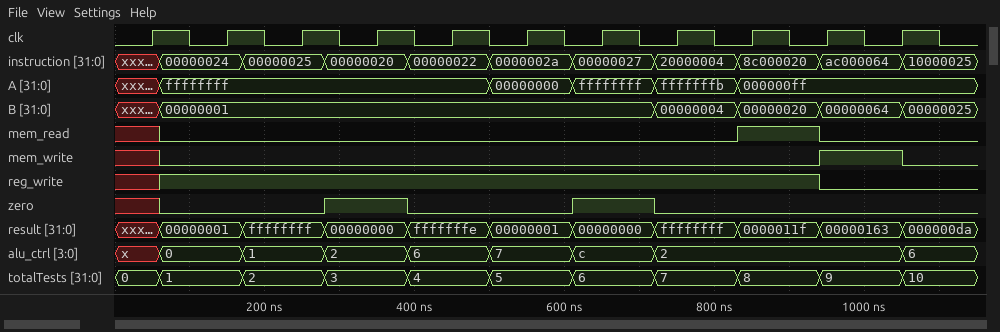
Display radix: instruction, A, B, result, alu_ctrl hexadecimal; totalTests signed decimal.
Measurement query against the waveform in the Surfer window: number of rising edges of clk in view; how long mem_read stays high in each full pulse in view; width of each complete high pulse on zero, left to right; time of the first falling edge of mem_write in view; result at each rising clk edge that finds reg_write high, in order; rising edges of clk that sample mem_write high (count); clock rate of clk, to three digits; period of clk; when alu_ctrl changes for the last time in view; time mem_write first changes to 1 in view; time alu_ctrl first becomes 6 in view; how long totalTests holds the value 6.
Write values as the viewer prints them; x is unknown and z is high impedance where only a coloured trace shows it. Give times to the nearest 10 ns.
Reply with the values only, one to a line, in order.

11
110 ns
110 ns, 110 ns
1050 ns
00000001, ffffffff, 00000000, fffffffe, 00000001, 00000000, ffffffff, 0000011f
2
10.0 MHz
100 ns
1050 ns
940 ns
390 ns
110 ns
